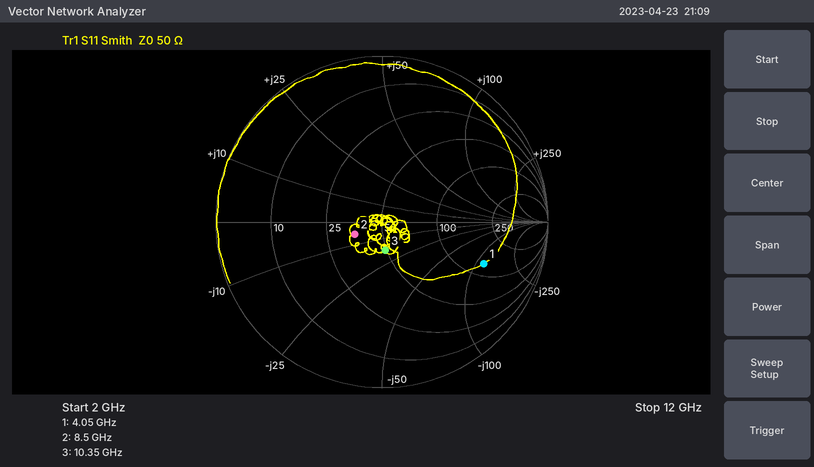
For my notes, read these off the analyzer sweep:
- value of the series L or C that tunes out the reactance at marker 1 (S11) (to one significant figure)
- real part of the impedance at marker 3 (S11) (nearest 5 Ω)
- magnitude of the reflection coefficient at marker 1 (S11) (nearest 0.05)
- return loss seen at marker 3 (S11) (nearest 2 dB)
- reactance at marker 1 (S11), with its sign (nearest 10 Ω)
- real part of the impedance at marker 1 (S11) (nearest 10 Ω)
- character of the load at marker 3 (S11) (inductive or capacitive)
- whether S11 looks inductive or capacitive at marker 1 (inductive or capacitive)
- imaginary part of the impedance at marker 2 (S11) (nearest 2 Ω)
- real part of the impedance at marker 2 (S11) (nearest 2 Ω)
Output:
5 nH
50 Ω
0.65
16 dB
-120 Ω
130 Ω
capacitive
capacitive
-6 Ω
36 Ω
